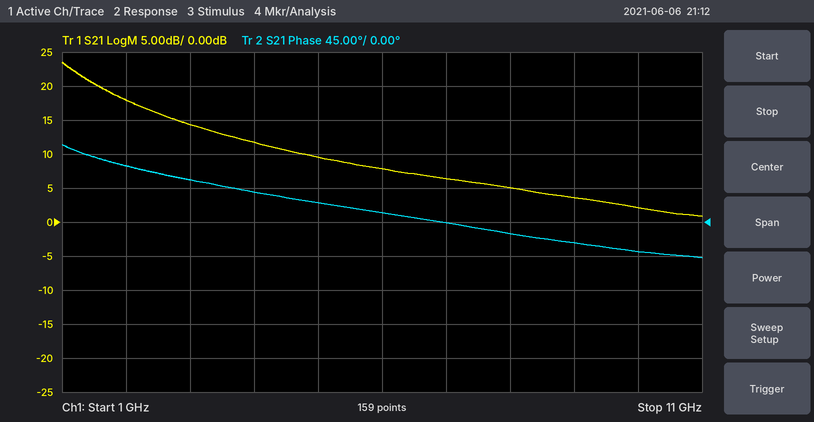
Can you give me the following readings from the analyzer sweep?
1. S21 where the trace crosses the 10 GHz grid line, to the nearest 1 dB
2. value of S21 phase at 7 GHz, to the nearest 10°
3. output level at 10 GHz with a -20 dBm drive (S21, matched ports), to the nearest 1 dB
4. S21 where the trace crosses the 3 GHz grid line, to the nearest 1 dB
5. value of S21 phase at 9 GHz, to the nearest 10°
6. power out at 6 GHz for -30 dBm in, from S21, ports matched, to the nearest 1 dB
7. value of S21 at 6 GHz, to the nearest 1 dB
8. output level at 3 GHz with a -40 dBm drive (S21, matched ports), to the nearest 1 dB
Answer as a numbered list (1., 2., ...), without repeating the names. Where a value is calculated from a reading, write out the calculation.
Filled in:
1. 2 dB
2. 0°
3. -20 dBm + (2 dB) = -18 dBm
4. 14 dB
5. -30°
6. -30 dBm + (8 dB) = -22 dBm
7. 8 dB
8. -40 dBm + (14 dB) = -26 dBm
